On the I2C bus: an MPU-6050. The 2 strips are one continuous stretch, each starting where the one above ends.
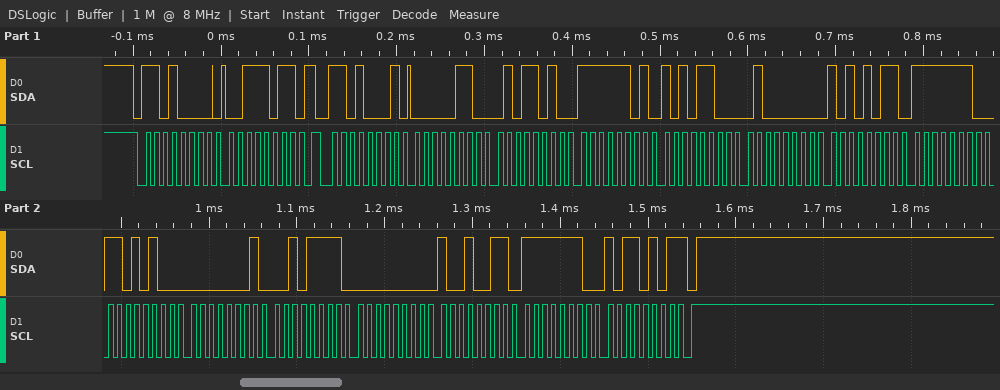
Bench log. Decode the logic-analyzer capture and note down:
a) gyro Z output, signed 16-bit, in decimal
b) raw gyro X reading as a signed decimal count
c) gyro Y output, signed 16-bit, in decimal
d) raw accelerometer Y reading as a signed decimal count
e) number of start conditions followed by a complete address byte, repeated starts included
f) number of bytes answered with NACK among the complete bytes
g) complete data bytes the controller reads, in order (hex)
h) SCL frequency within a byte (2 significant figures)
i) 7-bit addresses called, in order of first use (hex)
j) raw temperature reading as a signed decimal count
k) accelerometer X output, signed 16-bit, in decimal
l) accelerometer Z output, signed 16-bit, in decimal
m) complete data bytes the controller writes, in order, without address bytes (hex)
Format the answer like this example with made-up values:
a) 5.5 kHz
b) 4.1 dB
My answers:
a) -331
b) 303
c) 147
d) -596
e) 2
f) 1
g) 06 5A FD AC 40 AB FE D4 01 2F 00 93 FE B5
h) 100 kHz
i) 0x68
j) -300
k) 1626
l) 16555
m) 3B
